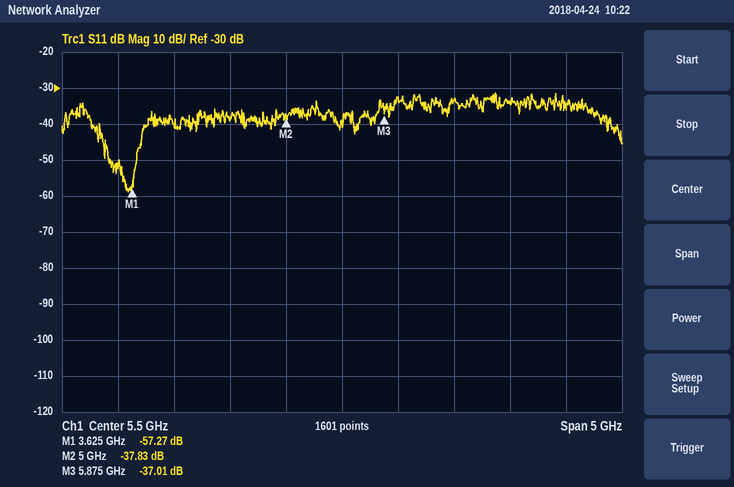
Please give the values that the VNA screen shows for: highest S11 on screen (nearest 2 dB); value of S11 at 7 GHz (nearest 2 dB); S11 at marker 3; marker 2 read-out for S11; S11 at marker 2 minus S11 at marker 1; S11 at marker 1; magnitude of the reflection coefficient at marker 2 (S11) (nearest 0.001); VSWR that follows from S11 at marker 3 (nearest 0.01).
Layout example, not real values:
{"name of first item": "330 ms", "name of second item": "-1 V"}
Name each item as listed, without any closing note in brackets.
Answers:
{"highest S11 on screen": "-32 dB", "value of S11 at 7 GHz": "-34 dB", "S11 at marker 3": "-37.01 dB", "marker 2 read-out for S11": "-37.83 dB", "S11 at marker 2 minus S11 at marker 1": "19.44 dB", "S11 at marker 1": "-57.27 dB", "magnitude of the reflection coefficient at marker 2 (S11)": "0.013", "VSWR that follows from S11 at marker 3": "1.03"}
